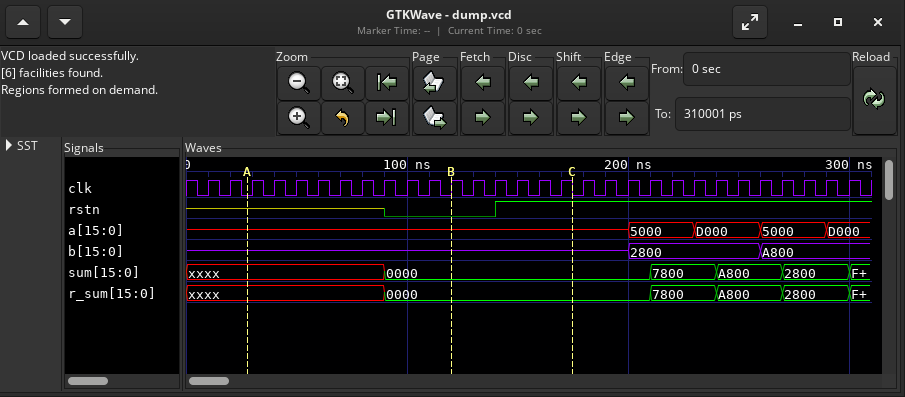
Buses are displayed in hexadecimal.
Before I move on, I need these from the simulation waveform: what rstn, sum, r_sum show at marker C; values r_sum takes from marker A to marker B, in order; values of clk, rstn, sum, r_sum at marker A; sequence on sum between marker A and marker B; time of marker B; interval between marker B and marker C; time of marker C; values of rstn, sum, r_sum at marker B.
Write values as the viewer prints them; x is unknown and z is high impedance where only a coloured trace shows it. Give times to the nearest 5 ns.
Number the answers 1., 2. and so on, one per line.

1. rstn=1, sum=0000, r_sum=0000
2. xxxx, 0000
3. clk=0, rstn=z, sum=xxxx, r_sum=xxxx
4. xxxx, 0000
5. 120 ns
6. 55 ns
7. 175 ns
8. rstn=0, sum=0000, r_sum=0000
